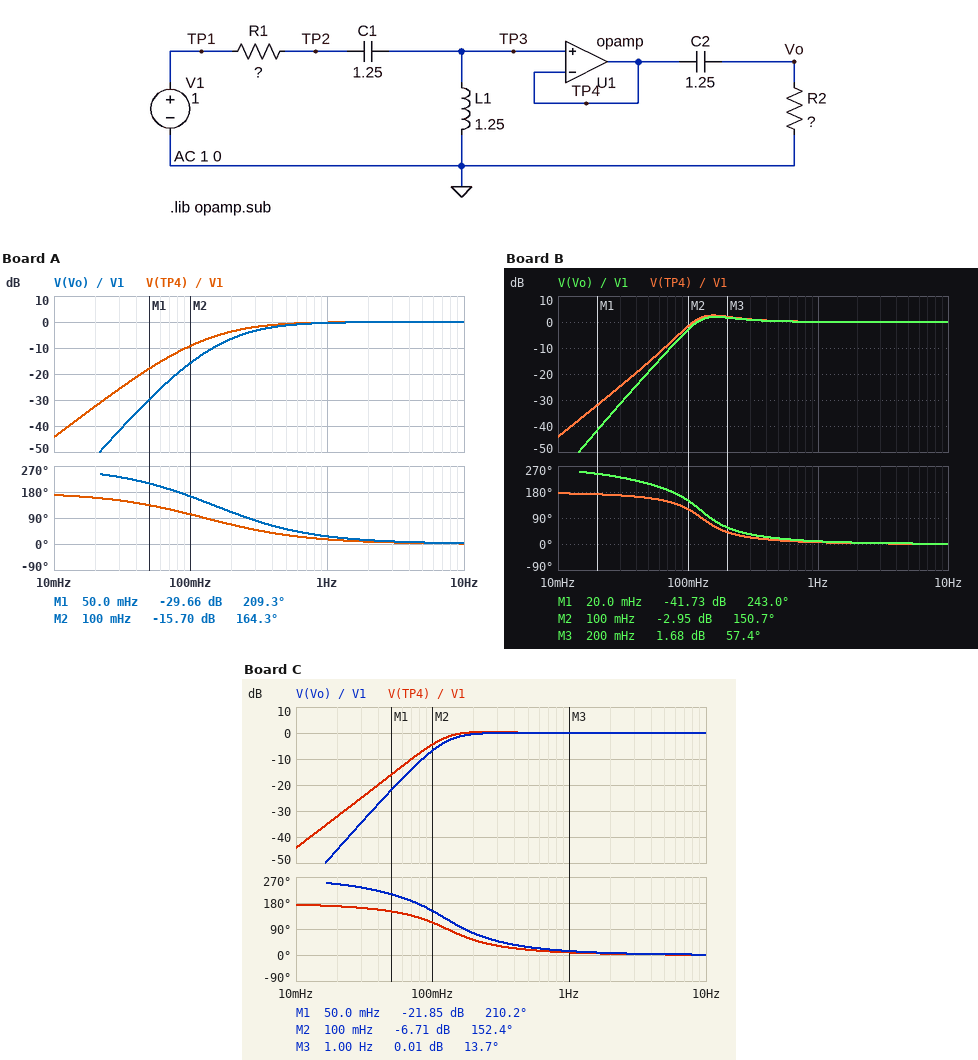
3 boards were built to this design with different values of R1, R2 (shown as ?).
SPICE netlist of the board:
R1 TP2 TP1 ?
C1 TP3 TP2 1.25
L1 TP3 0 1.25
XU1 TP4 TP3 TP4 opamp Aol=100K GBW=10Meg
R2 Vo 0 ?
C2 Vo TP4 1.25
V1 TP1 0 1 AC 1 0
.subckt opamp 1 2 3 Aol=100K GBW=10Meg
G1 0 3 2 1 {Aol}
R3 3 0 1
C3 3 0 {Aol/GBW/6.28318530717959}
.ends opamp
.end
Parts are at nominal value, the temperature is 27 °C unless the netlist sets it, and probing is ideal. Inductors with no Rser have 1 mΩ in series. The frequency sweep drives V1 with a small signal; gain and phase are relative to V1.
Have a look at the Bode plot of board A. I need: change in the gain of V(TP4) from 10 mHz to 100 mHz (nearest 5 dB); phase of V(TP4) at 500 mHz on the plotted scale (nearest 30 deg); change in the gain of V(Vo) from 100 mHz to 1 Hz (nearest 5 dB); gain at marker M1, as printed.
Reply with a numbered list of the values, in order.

1. 35 dB
2. 30 deg
3. 15 dB
4. -29.66 dB
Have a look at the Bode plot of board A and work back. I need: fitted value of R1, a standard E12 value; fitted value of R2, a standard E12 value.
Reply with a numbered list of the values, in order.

1. 2.2 Ω
2. 0.68 Ω
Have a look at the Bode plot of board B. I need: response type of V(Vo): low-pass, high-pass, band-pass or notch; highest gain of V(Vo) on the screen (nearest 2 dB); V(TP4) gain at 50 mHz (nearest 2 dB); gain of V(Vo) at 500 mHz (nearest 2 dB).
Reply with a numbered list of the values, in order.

1. high-pass
2. 2 dB
3. -16 dB
4. 0 dB
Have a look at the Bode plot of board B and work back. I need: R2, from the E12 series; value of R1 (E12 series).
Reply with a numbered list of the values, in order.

1. 2.2 Ω
2. 0.82 Ω
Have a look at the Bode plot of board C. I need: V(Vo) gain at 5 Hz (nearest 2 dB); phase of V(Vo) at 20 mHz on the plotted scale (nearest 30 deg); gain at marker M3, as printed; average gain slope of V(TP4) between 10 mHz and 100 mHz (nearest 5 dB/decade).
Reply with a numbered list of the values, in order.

1. 0 dB
2. 240 deg
3. 0.01 dB
4. 40 dB/decade
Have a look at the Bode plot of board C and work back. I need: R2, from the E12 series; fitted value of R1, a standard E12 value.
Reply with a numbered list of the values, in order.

1. 1.5 Ω
2. 1.2 Ω
